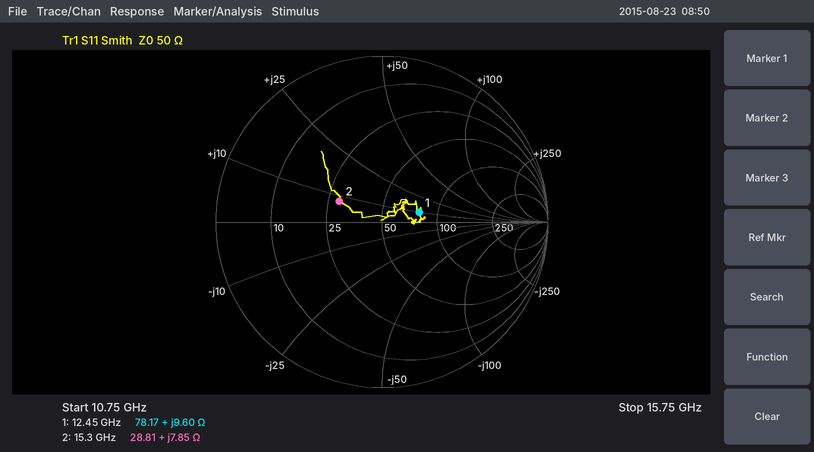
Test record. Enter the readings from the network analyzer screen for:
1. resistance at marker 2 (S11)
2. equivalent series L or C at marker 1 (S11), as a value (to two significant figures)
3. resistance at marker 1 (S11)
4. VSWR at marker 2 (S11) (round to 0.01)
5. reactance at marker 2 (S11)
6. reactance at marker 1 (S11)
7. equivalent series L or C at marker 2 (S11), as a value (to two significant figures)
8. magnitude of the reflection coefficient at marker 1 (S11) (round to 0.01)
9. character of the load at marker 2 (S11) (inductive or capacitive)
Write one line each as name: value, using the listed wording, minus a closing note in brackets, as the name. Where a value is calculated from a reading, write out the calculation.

resistance at marker 2: 28.81 Ω
equivalent series L or C at marker 1 (S11), as a value: L = 9.6 Ω/(2π × 12.45 GHz) ≈ 123 pH, so 120 pH to two significant figures
resistance at marker 1: 78.17 Ω
VSWR at marker 2 (S11): 1.80
reactance at marker 2: +7.85 Ω
reactance at marker 1: +9.60 Ω
equivalent series L or C at marker 2 (S11), as a value: L = 7.85 Ω/(2π × 15.3 GHz) ≈ 82 pH
magnitude of the reflection coefficient at marker 1 (S11): 0.23
character of the load at marker 2 (S11): inductive
